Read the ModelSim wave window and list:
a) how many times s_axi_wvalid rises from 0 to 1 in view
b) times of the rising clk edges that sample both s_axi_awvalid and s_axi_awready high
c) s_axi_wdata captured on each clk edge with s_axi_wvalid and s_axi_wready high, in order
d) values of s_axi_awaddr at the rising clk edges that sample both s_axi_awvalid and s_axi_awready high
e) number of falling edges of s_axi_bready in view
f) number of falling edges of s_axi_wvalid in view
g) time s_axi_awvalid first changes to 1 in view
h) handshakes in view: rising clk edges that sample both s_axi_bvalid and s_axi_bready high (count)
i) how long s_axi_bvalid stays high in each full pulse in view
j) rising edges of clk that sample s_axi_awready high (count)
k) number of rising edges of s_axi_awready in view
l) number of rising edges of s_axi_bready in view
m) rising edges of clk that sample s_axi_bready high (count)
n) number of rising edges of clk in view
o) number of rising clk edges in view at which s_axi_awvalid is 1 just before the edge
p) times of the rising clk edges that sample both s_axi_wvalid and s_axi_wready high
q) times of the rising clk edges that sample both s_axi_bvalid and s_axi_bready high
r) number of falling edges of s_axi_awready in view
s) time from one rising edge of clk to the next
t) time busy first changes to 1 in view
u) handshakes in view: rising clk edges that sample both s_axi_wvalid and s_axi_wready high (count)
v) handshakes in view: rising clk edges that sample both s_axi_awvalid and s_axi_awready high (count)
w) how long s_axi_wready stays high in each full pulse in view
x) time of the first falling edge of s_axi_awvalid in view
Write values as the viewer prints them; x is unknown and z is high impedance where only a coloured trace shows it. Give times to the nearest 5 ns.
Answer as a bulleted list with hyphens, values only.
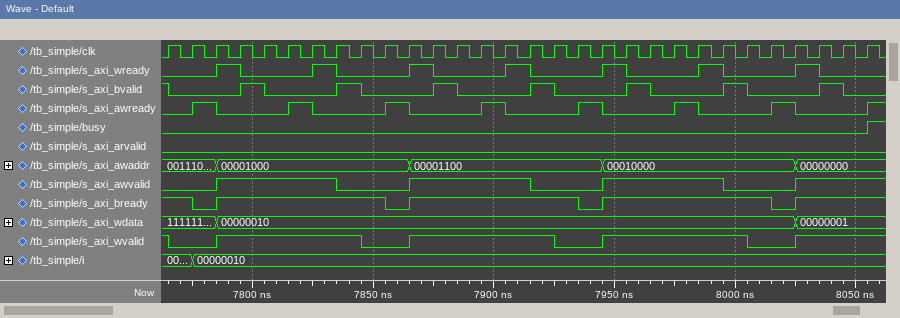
- 4
- 7825 ns, 7905 ns, 7985 ns
- 00000010, 00000010, 00000010, 00000010, 00000010, 00000010, 00000001
- 00001000, 00001100, 00010000
- 4
- 4
- 7785 ns
- 8
- 10 ns, 10 ns, 10 ns, 10 ns, 10 ns, 10 ns, 10 ns
- 7
- 8
- 4
- 26
- 30
- 18
- 7795 ns, 7835 ns, 7875 ns, 7915 ns, 7955 ns, 7995 ns, 8035 ns
- 7765 ns, 7805 ns, 7845 ns, 7885 ns, 7925 ns, 7965 ns, 8005 ns, 8045 ns
- 7
- 10 ns
- 8055 ns
- 7
- 3
- 10 ns, 10 ns, 10 ns, 10 ns, 10 ns, 10 ns, 10 ns
- 7835 ns
